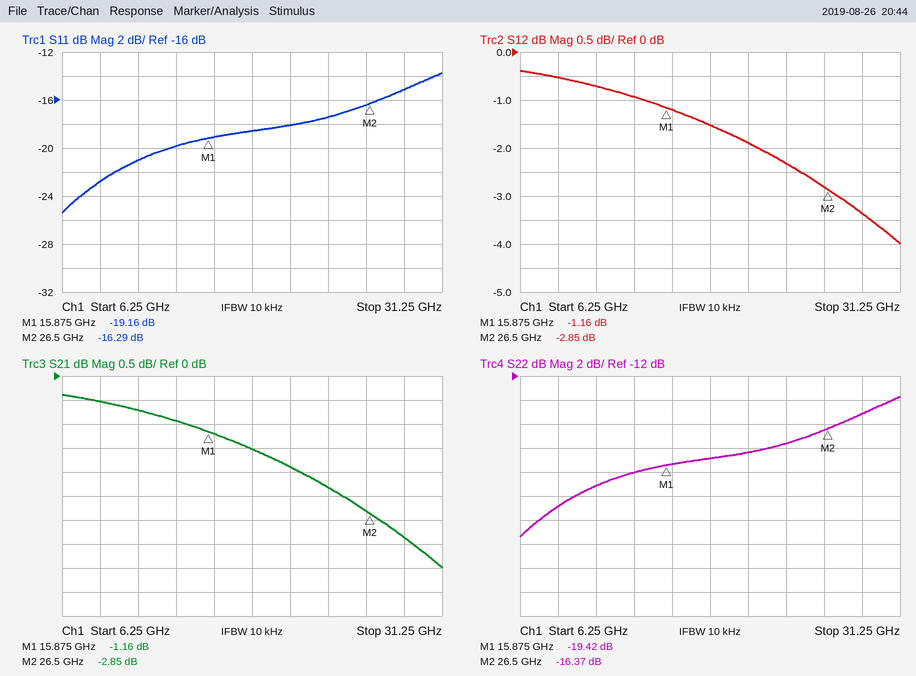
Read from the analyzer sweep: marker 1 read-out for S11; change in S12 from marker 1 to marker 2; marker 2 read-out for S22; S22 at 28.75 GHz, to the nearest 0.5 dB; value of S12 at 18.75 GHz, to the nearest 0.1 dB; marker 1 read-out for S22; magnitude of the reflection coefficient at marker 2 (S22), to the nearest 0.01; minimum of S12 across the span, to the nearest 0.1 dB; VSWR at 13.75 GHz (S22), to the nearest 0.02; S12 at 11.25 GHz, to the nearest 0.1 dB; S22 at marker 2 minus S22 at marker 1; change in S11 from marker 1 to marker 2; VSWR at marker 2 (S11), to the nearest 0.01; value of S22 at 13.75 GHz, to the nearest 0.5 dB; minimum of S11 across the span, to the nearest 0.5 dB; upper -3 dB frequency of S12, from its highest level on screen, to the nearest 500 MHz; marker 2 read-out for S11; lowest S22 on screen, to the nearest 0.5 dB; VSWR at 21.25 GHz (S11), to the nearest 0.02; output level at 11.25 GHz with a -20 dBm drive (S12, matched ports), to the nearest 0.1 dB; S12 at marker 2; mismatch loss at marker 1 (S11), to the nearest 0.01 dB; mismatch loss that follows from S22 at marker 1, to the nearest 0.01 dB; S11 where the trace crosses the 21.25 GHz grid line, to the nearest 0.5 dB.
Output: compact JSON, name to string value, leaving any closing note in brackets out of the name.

{"marker 1 read-out for S11": "-19.16 dB", "change in S12 from marker 1 to marker 2": "-1.69 dB", "marker 2 read-out for S22": "-16.37 dB", "S22 at 28.75 GHz, to the nearest 0.5 dB": "-15.0 dB", "value of S12 at 18.75 GHz, to the nearest 0.1 dB": "-1.5 dB", "marker 1 read-out for S22": "-19.42 dB", "magnitude of the reflection coefficient at marker 2 (S22), to the nearest 0.01": "0.15", "minimum of S12 across the span, to the nearest 0.1 dB": "-4.0 dB", "VSWR at 13.75 GHz (S22), to the nearest 0.02": "1.22", "S12 at 11.25 GHz, to the nearest 0.1 dB": "-0.7 dB", "S22 at marker 2 minus S22 at marker 1": "3.05 dB", "change in S11 from marker 1 to marker 2": "2.87 dB", "VSWR at marker 2 (S11), to the nearest 0.01": "1.36", "value of S22 at 13.75 GHz, to the nearest 0.5 dB": "-20.0 dB", "minimum of S11 across the span, to the nearest 0.5 dB": "-25.5 dB", "upper -3 dB frequency of S12, from its highest level on screen, to the nearest 500 MHz": "29.0 GHz", "marker 2 read-out for S11": "-16.29 dB", "lowest S22 on screen, to the nearest 0.5 dB": "-25.5 dB", "VSWR at 21.25 GHz (S11), to the nearest 0.02": "1.28", "output level at 11.25 GHz with a -20 dBm drive (S12, matched ports), to the nearest 0.1 dB": "-20.7 dBm", "S12 at marker 2": "-2.85 dB", "mismatch loss at marker 1 (S11), to the nearest 0.01 dB": "0.05 dB", "mismatch loss that follows from S22 at marker 1, to the nearest 0.01 dB": "0.05 dB", "S11 where the trace crosses the 21.25 GHz grid line, to the nearest 0.5 dB": "-18.0 dB"}
